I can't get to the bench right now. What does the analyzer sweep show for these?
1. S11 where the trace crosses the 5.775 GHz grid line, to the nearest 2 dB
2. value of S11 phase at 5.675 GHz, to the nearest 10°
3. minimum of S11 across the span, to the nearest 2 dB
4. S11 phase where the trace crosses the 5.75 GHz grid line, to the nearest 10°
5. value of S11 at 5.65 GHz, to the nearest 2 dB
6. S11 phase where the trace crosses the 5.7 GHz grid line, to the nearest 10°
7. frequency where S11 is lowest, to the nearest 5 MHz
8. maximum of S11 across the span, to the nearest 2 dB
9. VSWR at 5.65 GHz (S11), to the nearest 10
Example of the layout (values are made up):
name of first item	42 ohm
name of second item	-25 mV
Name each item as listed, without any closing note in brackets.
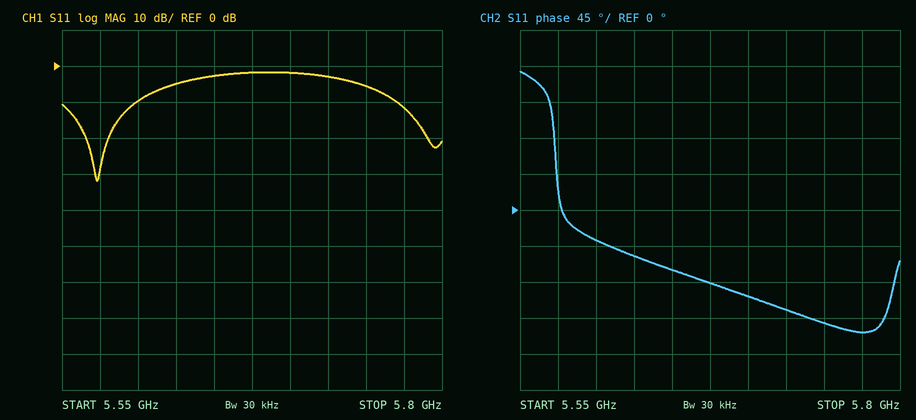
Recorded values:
S11 where the trace crosses the 5.775 GHz grid line, to the nearest 2 dB	-12 dB
value of S11 phase at 5.675 GHz, to the nearest 10°	-90°
minimum of S11 across the span, to the nearest 2 dB	-32 dB
S11 phase where the trace crosses the 5.75 GHz grid line, to the nearest 10°	-140°
value of S11 at 5.65 GHz, to the nearest 2 dB	-2 dB
S11 phase where the trace crosses the 5.7 GHz grid line, to the nearest 10°	-110°
frequency where S11 is lowest, to the nearest 5 MHz	5.575 GHz
maximum of S11 across the span, to the nearest 2 dB	-2 dB
VSWR at 5.65 GHz (S11), to the nearest 10	10
